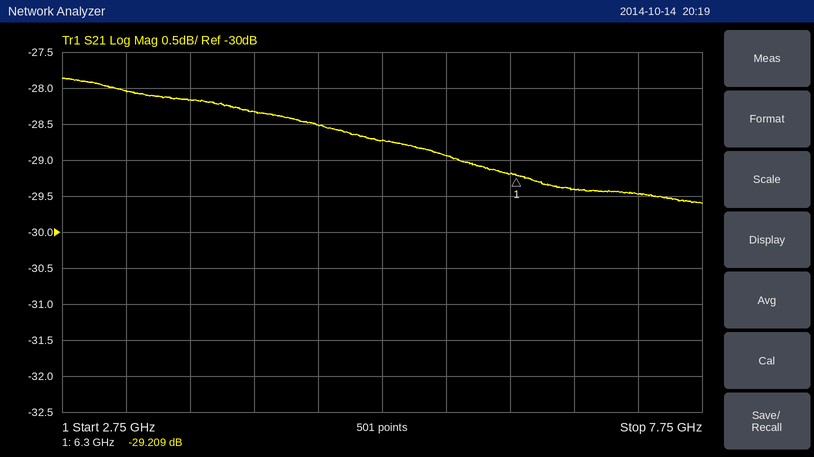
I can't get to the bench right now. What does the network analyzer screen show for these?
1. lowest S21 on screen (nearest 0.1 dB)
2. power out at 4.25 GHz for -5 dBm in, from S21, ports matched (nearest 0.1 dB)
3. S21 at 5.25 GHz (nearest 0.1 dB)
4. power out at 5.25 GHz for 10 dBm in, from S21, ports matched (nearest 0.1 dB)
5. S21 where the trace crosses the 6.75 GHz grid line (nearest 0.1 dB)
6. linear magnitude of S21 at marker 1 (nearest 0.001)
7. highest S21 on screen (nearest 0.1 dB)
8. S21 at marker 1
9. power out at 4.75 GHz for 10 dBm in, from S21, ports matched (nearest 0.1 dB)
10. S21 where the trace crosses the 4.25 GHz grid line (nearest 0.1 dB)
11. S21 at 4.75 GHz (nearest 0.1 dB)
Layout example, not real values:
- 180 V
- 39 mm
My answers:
- -29.6 dB
- -33.3 dBm
- -28.7 dB
- -18.7 dBm
- -29.4 dB
- 0.035
- -27.9 dB
- -29.209 dB
- -18.5 dBm
- -28.3 dB
- -28.5 dB
